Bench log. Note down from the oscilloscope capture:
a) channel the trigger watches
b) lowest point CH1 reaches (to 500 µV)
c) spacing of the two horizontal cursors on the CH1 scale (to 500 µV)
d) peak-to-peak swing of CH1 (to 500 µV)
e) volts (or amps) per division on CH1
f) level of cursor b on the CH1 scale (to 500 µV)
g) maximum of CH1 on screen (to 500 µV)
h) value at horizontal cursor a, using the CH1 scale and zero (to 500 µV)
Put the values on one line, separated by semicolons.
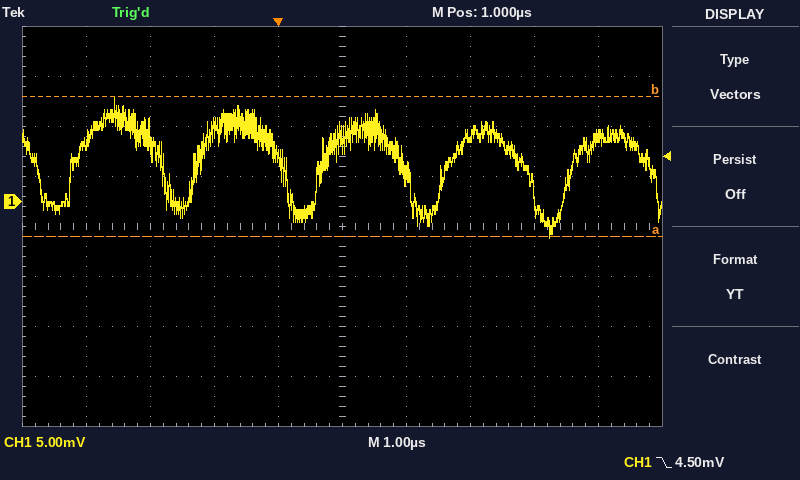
CH1; -3.5 mV; 14.0 mV; 14.0 mV; 5 mV; 10.5 mV; 10.5 mV; -3.5 mV
